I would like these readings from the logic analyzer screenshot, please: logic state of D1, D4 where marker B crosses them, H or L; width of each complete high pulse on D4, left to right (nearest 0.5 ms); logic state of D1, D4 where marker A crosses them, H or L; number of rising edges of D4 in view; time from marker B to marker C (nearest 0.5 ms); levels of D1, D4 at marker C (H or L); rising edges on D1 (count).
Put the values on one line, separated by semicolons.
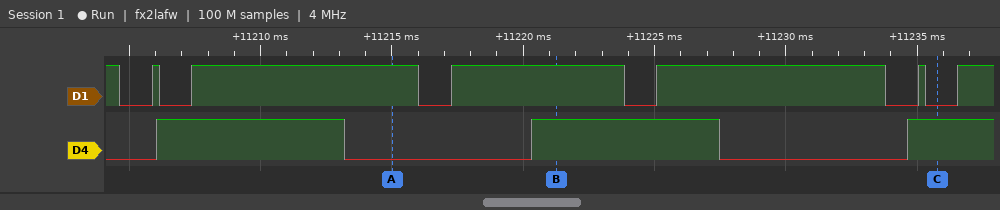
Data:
D1=H, D4=H; 7 ms, 7 ms; D1=H, D4=L; 3; 14.5 ms; D1=L, D4=H; 6
